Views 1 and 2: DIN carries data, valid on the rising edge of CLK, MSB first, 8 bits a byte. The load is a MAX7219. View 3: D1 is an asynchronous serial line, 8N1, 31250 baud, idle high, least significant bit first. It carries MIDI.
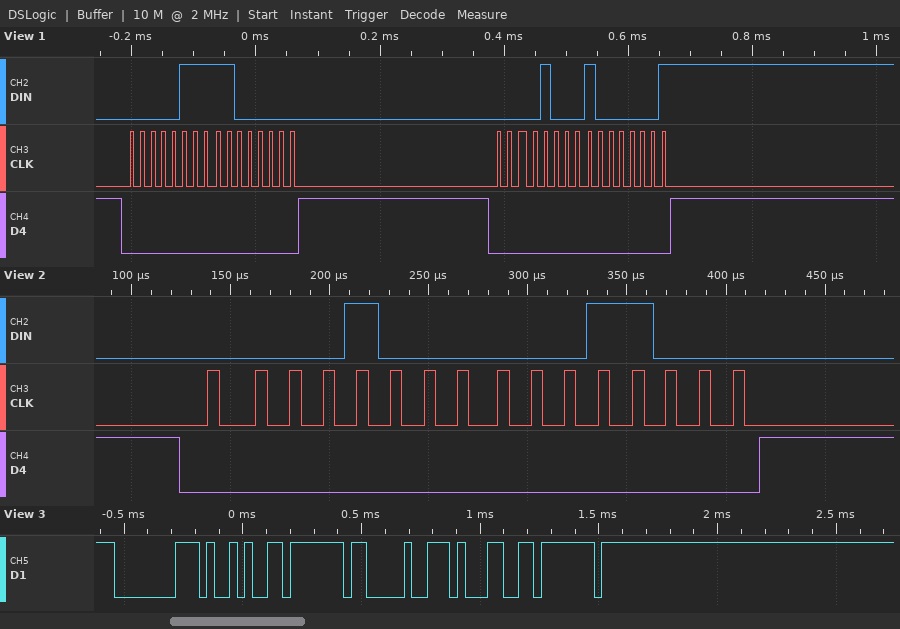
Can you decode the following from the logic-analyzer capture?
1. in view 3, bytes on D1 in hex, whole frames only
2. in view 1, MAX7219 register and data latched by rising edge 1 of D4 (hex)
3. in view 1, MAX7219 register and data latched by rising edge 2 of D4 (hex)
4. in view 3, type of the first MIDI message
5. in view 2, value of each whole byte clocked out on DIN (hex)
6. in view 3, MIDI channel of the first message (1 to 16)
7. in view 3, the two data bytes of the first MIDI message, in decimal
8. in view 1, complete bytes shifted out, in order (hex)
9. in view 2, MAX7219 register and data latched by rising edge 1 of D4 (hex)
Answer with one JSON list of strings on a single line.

["80 29 7F 90 31 7F", "register 0x7, data 0xC0", "register 0x8, data 0x81", "Note Off", "08 18", "1", "41, 127", "0x07 0xC0 0x08 0x81", "register 0x8, data 0x18"]
